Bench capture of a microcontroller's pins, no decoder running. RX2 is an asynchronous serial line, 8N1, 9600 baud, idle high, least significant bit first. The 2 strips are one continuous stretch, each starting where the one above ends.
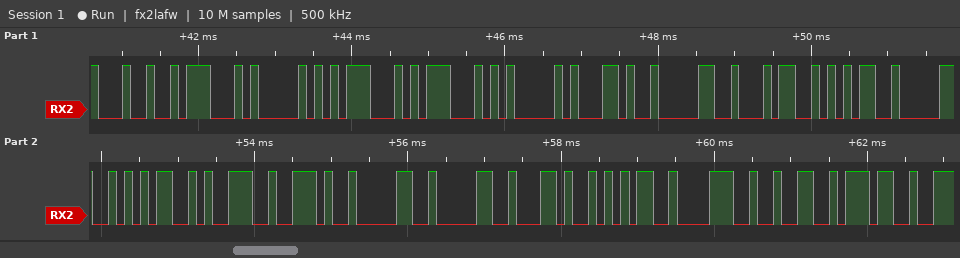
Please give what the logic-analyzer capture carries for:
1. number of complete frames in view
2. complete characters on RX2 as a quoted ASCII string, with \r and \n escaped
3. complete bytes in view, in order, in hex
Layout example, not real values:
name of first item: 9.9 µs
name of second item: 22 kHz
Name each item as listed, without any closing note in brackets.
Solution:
number of complete frames in view: 21
complete characters on RX2 as a quoted ASCII string, with \r and \n escaped: "$GPGGA,045059.00,5827"
complete bytes in view, in order, in hex: 24 47 50 47 47 41 2C 30 34 35 30 35 39 2E 30 30 2C 35 38 32 37
